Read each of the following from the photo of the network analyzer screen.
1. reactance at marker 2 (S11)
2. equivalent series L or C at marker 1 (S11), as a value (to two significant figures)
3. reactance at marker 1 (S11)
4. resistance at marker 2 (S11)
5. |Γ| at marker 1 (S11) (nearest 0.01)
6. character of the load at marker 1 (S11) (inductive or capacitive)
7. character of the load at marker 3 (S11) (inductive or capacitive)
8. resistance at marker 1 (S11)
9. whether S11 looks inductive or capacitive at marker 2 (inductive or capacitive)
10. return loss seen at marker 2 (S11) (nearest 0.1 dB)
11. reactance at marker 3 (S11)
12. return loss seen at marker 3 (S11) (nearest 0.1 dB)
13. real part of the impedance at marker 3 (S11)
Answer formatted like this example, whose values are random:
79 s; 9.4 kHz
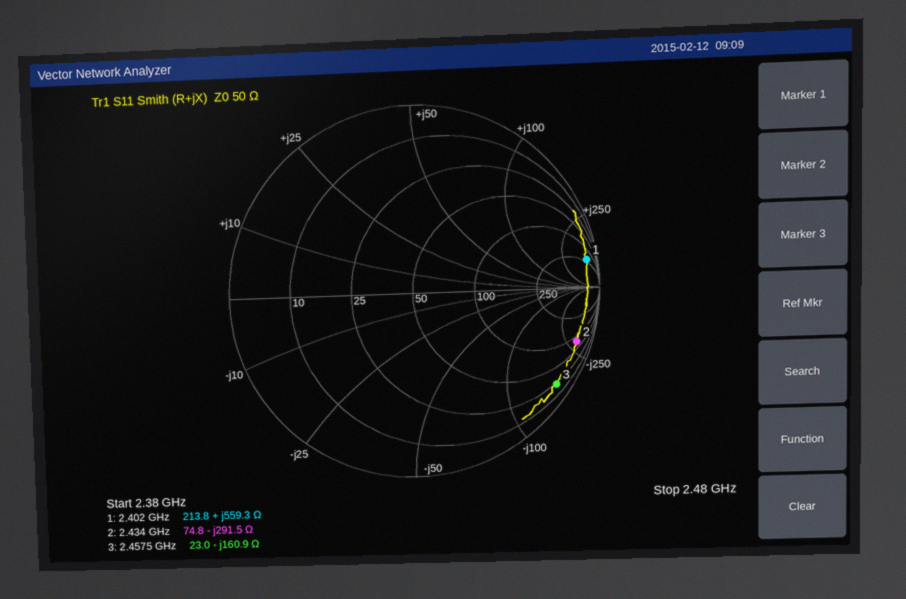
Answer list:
-291.5 Ω; 37 nH; +559.3 Ω; 74.8 Ω; 0.94; inductive; capacitive; 213.8 Ω; capacitive; 0.7 dB; -160.9 Ω; 0.7 dB; 23.0 Ω
